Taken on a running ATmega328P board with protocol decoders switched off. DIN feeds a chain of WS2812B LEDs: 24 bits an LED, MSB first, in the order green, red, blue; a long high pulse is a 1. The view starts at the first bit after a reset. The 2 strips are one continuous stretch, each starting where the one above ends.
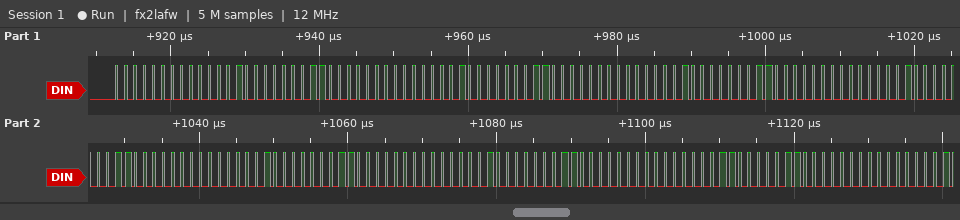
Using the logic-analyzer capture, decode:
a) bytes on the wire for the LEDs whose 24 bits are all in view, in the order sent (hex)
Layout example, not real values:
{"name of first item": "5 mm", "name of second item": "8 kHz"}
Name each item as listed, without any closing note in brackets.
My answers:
{"bytes on the wire for the LEDs whose 24 bits are all in view, in the order sent": "00 04 06 00 04 06 00 04 06 00 04 06 00 04 06 00 04 06 00 03 06"}
